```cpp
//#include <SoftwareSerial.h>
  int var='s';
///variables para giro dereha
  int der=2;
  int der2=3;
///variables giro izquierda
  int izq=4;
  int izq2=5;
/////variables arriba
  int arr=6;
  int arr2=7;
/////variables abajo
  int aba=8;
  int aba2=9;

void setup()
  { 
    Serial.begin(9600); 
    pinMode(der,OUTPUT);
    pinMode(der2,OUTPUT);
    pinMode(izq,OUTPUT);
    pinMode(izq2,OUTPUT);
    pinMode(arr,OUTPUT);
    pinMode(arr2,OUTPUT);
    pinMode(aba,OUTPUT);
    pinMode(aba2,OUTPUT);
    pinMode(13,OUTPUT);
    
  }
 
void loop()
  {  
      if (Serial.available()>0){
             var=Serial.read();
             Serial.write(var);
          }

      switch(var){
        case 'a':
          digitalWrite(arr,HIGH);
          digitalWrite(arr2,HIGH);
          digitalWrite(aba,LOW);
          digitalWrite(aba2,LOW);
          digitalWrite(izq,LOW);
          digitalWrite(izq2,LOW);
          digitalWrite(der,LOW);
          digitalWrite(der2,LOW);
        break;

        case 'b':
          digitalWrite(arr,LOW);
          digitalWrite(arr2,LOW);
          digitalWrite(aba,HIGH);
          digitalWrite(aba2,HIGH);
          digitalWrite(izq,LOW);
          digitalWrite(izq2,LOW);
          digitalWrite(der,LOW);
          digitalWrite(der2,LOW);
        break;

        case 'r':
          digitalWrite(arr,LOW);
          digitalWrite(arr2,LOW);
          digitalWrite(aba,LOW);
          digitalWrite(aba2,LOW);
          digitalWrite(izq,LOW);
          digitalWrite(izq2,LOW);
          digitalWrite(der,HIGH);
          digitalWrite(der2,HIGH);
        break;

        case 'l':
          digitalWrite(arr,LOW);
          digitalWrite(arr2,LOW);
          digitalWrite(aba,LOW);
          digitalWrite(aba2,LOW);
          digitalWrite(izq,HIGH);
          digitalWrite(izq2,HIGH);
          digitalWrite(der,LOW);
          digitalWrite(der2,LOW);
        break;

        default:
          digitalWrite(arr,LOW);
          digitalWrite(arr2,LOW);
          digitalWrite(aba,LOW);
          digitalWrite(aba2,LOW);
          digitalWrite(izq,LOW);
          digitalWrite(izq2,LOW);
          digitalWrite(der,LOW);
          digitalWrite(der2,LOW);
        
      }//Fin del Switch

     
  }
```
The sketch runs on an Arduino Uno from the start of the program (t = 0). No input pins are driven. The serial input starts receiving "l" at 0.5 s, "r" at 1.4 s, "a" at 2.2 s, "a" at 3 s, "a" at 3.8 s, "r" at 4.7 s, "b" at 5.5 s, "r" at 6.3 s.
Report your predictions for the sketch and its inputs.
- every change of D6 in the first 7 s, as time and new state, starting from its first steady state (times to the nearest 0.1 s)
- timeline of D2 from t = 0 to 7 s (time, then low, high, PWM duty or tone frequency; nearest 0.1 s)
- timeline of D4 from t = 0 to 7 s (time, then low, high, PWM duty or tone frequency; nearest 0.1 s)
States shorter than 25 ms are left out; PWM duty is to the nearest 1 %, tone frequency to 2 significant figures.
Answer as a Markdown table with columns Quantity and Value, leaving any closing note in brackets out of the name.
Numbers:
| Quantity | Value |
|---|---|
| every change of D6 in the first 7 s, as time and new state, starting from its first steady state | 0 s low; 2.2 s high; 4.7 s low |
| timeline of D2 from t = 0 to 7 s | 0 s low; 1.4 s high; 2.2 s low; 4.7 s high; 5.5 s low; 6.3 s high |
| timeline of D4 from t = 0 to 7 s | 0 s low; 0.5 s high; 1.4 s low |
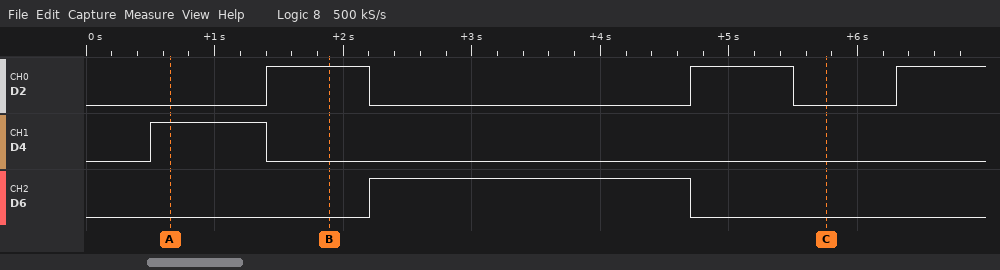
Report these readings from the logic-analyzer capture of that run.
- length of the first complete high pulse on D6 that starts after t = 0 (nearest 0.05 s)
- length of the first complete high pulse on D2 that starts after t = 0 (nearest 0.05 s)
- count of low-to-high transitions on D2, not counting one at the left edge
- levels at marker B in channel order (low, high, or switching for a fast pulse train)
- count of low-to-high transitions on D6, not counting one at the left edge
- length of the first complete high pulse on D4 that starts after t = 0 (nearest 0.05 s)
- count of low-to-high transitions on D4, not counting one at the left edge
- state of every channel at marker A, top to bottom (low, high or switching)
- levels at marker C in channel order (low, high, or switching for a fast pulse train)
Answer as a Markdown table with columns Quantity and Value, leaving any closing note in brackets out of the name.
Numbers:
| Quantity | Value |
|---|---|
| length of the first complete high pulse on D6 that starts after t = 0 | 2.50 s |
| length of the first complete high pulse on D2 that starts after t = 0 | 0.80 s |
| count of low-to-high transitions on D2, not counting one at the left edge | 3 |
| levels at marker B in channel order | D2 high, D4 low, D6 low |
| count of low-to-high transitions on D6, not counting one at the left edge | 1 |
| length of the first complete high pulse on D4 that starts after t = 0 | 0.90 s |
| count of low-to-high transitions on D4, not counting one at the left edge | 1 |
| state of every channel at marker A, top to bottom | D2 low, D4 high, D6 low |
| levels at marker C in channel order | D2 low, D4 low, D6 low |
